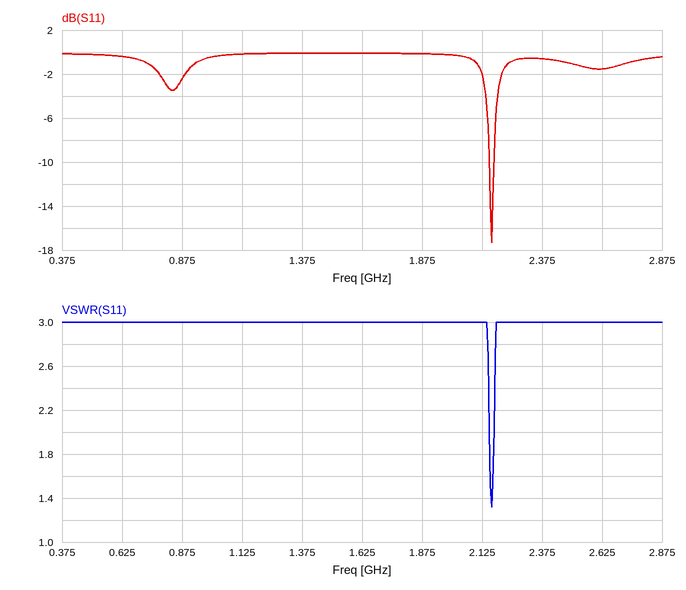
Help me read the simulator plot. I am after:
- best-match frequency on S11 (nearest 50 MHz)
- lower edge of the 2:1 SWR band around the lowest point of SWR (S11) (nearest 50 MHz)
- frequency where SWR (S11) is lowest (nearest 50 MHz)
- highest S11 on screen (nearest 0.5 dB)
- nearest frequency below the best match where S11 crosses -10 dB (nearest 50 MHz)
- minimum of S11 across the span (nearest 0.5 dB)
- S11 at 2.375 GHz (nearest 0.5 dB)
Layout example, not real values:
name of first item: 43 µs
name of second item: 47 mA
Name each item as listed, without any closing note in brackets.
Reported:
best-match frequency on S11: 2.15 GHz
lower edge of the 2:1 SWR band around the lowest point of SWR (S11): 2.15 GHz
frequency where SWR (S11) is lowest: 2.15 GHz
highest S11 on screen: 0.0 dB
nearest frequency below the best match where S11 crosses -10 dB: 2.15 GHz
minimum of S11 across the span: -17.5 dB
S11 at 2.375 GHz: -0.5 dB
